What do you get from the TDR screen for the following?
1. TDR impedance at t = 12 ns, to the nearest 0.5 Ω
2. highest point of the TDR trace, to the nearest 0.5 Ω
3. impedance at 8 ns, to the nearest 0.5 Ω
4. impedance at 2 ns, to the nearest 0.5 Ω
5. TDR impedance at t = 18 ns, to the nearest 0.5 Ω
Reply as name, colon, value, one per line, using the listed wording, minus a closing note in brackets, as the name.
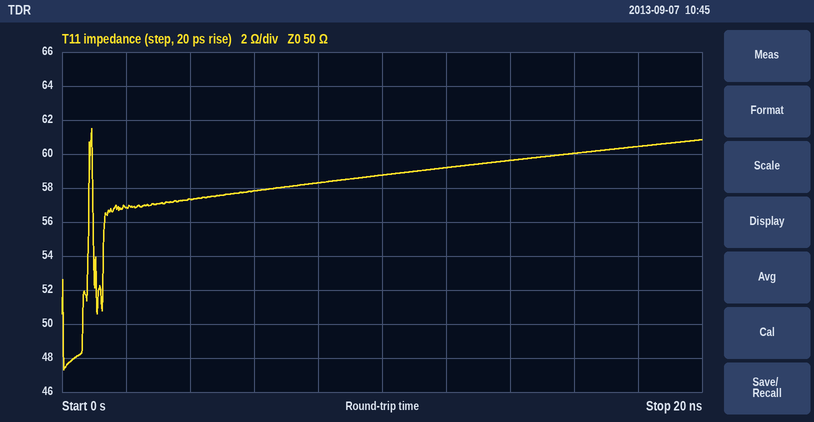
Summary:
TDR impedance at t = 12 ns, to the nearest 0.5 Ω: 59.0 Ω
highest point of the TDR trace, to the nearest 0.5 Ω: 61.5 Ω
impedance at 8 ns, to the nearest 0.5 Ω: 58.5 Ω
impedance at 2 ns, to the nearest 0.5 Ω: 57.0 Ω
TDR impedance at t = 18 ns, to the nearest 0.5 Ω: 60.5 Ω
